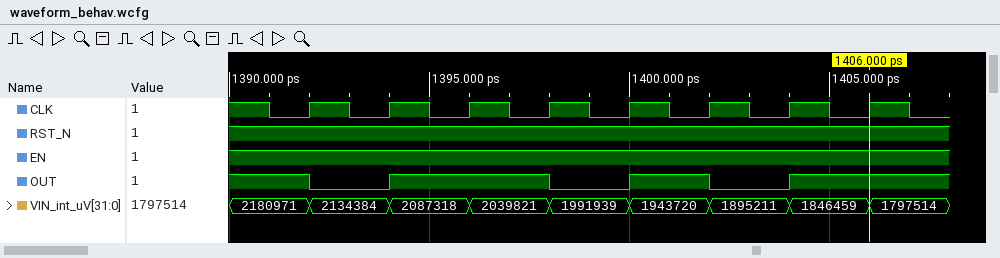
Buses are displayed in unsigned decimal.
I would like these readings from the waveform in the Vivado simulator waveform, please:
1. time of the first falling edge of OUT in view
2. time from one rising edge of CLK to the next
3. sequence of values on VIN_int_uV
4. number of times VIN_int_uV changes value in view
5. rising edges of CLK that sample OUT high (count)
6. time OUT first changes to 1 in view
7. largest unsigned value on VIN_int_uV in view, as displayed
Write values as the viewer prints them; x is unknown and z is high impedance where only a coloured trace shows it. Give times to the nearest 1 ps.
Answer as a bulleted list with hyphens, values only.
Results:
- 1392 ps
- 2 ps
- 2180971, 2134384, 2087318, 2039821, 1991939, 1943720, 1895211, 1846459, 1797514
- 8
- 5
- 1394 ps
- 2180971
